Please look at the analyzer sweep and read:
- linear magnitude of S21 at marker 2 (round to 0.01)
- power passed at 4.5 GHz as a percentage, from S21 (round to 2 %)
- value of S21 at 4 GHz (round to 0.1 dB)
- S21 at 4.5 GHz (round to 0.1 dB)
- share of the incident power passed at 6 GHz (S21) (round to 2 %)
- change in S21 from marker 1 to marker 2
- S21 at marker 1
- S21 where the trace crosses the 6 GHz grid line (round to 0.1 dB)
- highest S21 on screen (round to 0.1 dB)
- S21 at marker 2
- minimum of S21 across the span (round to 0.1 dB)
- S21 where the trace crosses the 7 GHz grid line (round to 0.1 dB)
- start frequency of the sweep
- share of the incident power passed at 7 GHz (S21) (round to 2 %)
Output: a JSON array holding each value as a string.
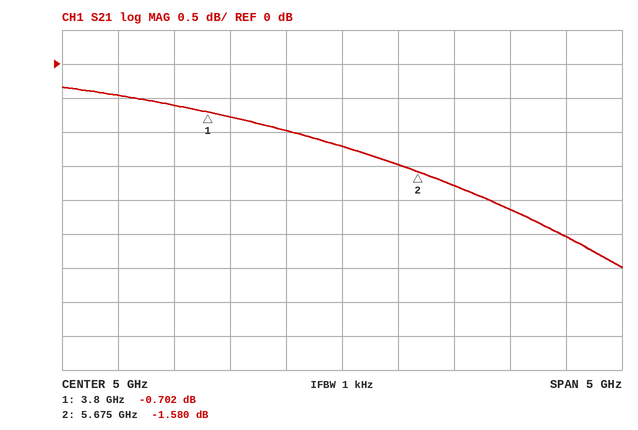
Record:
["0.83", "80 %", "-0.8 dB", "-1.0 dB", "66 %", "-0.878 dB", "-0.702 dB", "-1.8 dB", "-0.3 dB", "-1.580 dB", "-3.0 dB", "-2.5 dB", "2.5 GHz", "56 %"]
